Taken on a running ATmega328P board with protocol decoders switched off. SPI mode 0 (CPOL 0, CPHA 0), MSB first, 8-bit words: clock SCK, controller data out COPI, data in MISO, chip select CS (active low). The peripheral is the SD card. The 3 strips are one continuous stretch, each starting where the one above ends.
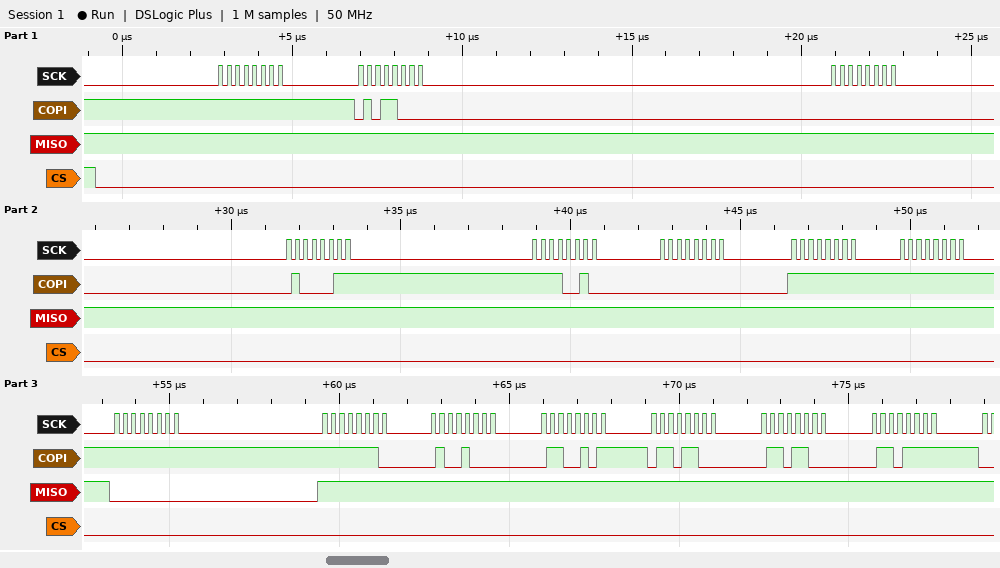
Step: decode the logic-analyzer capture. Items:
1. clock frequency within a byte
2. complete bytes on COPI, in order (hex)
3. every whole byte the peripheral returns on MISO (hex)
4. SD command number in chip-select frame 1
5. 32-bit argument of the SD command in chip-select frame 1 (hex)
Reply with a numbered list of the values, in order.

1. 4 MHz
2. FF 58 00 43 F2 00 FF FF FF FE 48 65 6C 6C 6F
3. FF FF FF FF FF FF FF FF 00 FF FF FF FF FF FF
4. CMD24
5. 0x0043F200
